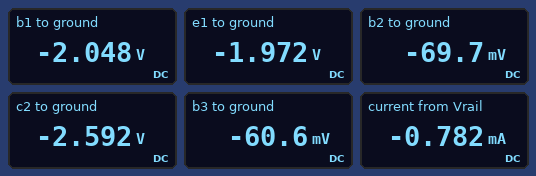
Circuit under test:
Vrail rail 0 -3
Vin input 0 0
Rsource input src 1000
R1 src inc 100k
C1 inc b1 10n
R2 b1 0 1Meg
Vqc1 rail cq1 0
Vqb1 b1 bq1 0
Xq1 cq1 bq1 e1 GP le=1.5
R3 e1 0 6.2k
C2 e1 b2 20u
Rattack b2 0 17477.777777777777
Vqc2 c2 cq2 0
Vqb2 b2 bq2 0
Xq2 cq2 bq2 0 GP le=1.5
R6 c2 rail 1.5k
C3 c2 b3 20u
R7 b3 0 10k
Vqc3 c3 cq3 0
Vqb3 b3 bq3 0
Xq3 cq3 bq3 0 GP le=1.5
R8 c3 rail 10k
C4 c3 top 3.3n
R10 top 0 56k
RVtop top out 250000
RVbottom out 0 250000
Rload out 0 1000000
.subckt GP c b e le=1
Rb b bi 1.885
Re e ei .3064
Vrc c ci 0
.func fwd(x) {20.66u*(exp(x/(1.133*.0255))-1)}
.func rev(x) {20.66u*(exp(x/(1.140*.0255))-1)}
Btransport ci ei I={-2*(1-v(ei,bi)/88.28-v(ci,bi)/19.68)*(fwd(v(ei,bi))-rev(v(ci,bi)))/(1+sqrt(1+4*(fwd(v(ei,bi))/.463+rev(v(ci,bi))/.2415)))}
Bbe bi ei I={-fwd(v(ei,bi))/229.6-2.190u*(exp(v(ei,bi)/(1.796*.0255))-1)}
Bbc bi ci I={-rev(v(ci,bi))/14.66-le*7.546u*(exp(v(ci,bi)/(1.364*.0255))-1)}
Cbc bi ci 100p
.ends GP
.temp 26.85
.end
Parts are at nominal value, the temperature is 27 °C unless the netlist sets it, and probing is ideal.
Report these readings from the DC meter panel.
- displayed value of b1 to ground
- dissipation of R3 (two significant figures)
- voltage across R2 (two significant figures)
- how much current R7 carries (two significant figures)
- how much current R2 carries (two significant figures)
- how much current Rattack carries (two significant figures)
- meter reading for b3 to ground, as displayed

-2.048 V
630 µW
2.0 V
6.1 µA
2.0 µA
4.0 µA
-60.6 mV
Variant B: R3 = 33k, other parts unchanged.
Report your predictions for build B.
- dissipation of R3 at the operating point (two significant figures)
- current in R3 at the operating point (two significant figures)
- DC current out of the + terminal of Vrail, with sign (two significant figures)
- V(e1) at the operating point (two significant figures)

260 µW
89 µA
-550 µA
-2.9 V
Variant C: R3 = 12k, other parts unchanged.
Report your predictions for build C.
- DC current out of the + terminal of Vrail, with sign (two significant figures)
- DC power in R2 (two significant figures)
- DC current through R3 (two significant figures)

-700 µA
8.5 µW
240 µA
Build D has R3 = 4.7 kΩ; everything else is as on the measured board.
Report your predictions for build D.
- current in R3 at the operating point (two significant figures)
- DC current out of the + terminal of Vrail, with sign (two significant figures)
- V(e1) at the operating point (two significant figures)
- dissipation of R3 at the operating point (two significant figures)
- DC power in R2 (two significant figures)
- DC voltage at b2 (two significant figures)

340 µA
-800 µA
-1.6 V
540 µW
2.8 µW
-70 mV
